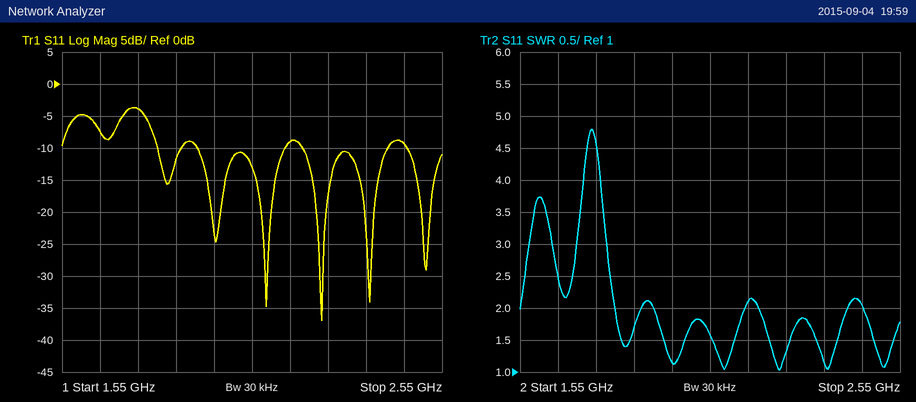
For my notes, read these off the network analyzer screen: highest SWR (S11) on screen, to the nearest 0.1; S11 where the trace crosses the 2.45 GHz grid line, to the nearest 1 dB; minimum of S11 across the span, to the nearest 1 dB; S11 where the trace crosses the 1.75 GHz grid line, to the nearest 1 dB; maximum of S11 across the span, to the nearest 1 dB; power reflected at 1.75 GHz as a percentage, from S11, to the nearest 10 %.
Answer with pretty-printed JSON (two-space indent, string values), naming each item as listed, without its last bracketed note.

{
  "highest SWR (S11) on screen, to the nearest 0.1": "4.8",
  "S11 where the trace crosses the 2.45 GHz grid line, to the nearest 1 dB": "-9 dB",
  "minimum of S11 across the span, to the nearest 1 dB": "-37 dB",
  "S11 where the trace crosses the 1.75 GHz grid line, to the nearest 1 dB": "-4 dB",
  "maximum of S11 across the span, to the nearest 1 dB": "-4 dB",
  "power reflected at 1.75 GHz as a percentage, from S11, to the nearest 10 %": "40 %"
}
